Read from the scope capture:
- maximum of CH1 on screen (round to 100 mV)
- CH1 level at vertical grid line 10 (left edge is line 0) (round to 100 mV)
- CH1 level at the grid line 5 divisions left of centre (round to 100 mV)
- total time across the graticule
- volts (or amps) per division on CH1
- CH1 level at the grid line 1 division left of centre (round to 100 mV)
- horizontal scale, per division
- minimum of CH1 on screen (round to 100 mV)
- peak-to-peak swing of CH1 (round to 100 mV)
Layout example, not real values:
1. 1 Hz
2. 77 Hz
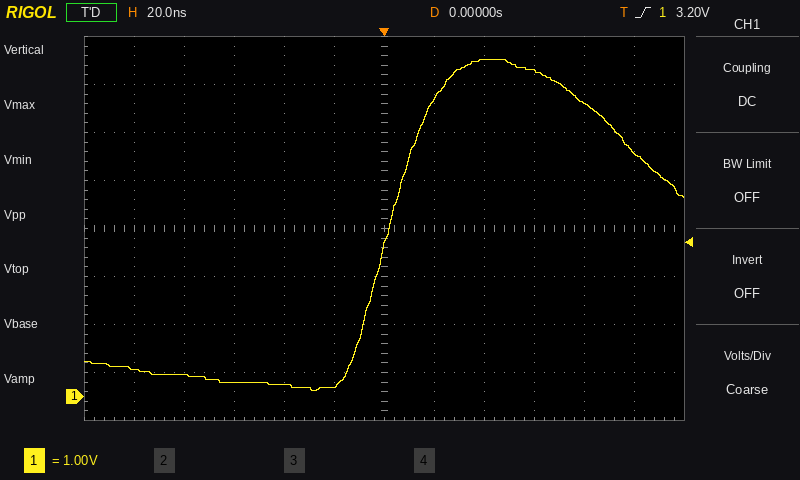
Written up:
1. 7.0 V
2. 6.1 V
3. 600 mV
4. 240 ns
5. 1 V
6. 200 mV
7. 20 ns
8. 100 mV
9. 6.9 V
